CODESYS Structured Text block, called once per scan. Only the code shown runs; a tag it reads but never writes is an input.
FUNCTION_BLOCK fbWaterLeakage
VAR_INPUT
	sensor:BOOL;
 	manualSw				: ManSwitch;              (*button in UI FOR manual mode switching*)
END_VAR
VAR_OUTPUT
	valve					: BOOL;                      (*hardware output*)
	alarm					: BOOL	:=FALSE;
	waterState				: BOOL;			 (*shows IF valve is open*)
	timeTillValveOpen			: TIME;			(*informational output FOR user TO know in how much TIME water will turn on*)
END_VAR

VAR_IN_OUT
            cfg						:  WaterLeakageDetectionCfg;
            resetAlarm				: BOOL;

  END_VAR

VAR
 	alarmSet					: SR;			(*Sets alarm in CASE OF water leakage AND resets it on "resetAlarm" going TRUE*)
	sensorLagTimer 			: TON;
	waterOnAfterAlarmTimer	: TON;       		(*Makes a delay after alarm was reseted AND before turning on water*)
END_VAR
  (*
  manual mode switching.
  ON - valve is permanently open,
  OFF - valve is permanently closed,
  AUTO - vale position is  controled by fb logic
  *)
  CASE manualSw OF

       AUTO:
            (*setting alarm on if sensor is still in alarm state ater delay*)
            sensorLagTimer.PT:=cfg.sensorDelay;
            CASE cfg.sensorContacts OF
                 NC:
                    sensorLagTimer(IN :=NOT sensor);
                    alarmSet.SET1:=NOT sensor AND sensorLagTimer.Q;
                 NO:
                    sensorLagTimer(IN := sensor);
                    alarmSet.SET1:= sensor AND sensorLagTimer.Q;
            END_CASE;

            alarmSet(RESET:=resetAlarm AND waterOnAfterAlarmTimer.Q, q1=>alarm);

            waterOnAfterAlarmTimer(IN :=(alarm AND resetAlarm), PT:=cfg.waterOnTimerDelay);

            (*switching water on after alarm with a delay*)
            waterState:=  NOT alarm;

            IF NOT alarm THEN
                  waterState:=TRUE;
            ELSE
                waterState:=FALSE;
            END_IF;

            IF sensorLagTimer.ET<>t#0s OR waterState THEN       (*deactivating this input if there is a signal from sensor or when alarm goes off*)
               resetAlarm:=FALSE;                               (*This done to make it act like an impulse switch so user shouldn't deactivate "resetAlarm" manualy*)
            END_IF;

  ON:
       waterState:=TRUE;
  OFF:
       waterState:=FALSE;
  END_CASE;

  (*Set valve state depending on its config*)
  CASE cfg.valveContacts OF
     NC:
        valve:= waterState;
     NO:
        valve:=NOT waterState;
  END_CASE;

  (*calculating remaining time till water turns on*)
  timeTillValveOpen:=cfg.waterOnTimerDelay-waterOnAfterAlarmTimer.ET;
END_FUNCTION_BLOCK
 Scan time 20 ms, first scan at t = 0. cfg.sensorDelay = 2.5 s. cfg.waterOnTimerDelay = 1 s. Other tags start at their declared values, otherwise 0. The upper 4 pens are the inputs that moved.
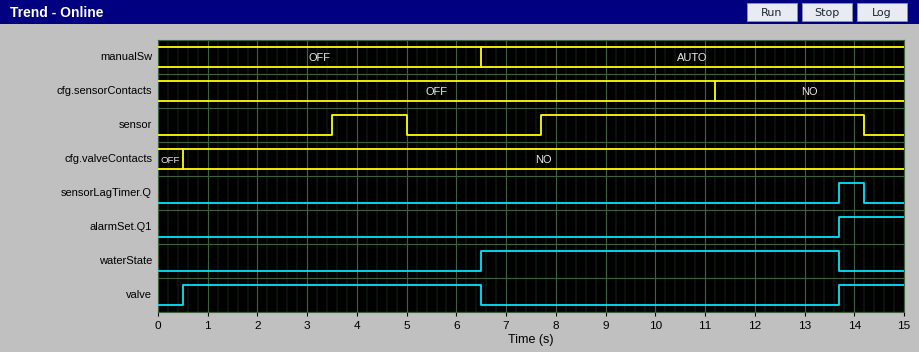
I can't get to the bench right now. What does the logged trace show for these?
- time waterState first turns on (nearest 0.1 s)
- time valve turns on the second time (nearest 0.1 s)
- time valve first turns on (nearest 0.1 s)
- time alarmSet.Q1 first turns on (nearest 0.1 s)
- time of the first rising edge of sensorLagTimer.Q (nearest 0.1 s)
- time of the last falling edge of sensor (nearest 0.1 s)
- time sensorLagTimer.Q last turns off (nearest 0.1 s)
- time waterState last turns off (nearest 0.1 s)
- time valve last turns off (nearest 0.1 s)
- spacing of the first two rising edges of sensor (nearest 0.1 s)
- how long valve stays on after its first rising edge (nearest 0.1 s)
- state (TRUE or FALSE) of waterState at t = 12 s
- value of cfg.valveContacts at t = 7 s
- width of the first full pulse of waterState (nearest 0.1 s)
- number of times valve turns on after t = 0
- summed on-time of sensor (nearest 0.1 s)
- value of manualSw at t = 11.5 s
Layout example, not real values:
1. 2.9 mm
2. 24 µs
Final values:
1. 6.5 s
2. 13.7 s
3. 0.5 s
4. 13.7 s
5. 13.7 s
6. 14.2 s
7. 14.2 s
8. 13.7 s
9. 6.5 s
10. 4.2 s
11. 6.0 s
12. TRUE
13. NO
14. 7.2 s
15. 2
16. 8.0 s
17. AUTO
